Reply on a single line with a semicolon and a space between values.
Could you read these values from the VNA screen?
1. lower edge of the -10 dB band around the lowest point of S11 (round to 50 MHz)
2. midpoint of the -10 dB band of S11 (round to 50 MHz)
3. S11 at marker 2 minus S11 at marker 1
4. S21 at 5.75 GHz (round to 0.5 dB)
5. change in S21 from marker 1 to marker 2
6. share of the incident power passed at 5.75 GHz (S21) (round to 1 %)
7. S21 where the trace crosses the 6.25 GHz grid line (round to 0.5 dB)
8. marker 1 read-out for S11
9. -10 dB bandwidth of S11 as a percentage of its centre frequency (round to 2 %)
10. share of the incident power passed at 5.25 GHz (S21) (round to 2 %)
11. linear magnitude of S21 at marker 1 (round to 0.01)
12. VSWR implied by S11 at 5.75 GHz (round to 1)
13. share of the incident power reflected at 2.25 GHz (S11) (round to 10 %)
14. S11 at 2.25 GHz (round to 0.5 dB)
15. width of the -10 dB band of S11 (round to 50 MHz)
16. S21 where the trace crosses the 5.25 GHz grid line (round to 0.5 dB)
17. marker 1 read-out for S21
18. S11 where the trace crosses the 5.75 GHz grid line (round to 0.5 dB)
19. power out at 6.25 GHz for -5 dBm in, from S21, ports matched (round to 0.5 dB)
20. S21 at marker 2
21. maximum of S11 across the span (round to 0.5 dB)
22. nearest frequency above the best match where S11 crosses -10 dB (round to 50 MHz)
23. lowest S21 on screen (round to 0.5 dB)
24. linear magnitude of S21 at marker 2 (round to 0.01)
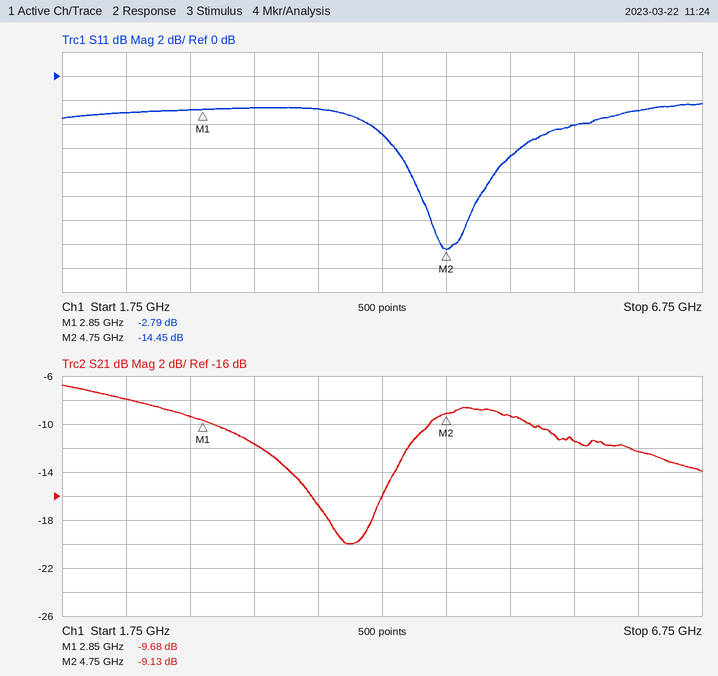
4.55 GHz; 4.80 GHz; -11.66 dB; -11.5 dB; 0.55 dB; 7 %; -12.5 dB; -2.79 dB; 10 %; 12 %; 0.33; 4; 50 %; -3.0 dB; 450 MHz; -9.5 dB; -9.68 dB; -4.0 dB; -17.5 dBm; -9.13 dB; -2.5 dB; 5.00 GHz; -20.0 dB; 0.35
